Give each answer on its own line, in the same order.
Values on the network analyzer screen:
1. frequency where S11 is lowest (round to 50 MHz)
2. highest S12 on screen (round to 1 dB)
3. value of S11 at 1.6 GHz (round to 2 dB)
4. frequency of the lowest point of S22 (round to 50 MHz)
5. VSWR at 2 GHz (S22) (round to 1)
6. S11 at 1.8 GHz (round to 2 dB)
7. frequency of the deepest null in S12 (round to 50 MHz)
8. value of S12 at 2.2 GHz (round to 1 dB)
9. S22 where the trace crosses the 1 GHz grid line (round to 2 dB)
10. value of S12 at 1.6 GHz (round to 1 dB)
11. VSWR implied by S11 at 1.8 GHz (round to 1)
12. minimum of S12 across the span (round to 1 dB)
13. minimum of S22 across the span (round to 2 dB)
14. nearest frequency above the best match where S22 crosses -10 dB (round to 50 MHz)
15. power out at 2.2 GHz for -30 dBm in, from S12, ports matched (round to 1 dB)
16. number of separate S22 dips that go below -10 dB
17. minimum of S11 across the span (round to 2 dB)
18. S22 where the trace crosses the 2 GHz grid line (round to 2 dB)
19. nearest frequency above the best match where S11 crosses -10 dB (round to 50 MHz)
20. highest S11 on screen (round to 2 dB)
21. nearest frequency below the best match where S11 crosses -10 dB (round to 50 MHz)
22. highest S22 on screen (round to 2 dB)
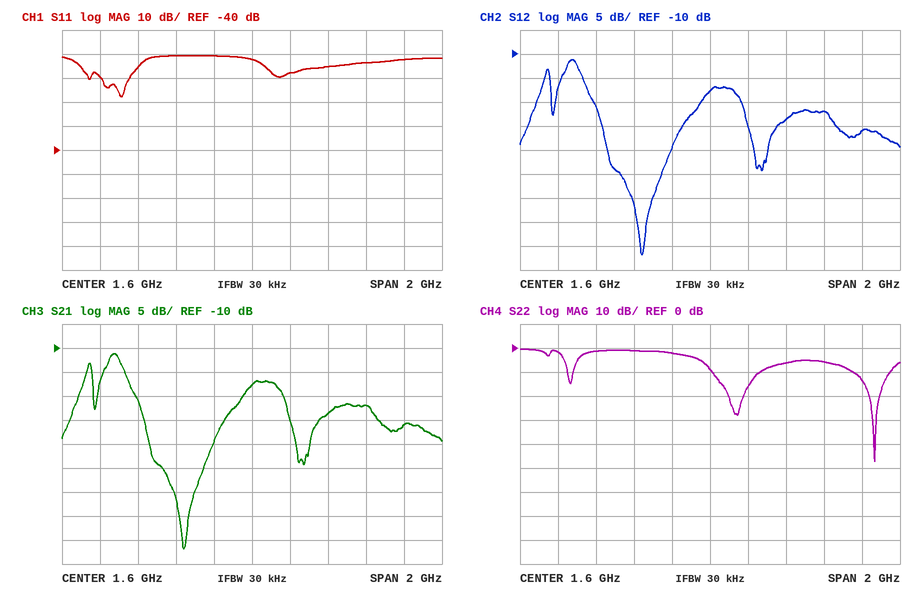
900 MHz
-11 dB
-2 dB
2.45 GHz
3
-8 dB
1.25 GHz
-22 dB
-2 dB
-18 dB
2
-52 dB
-48 dB
2.55 GHz
-52 dBm
3
-18 dB
-6 dB
950 MHz
0 dB
800 MHz
0 dB
